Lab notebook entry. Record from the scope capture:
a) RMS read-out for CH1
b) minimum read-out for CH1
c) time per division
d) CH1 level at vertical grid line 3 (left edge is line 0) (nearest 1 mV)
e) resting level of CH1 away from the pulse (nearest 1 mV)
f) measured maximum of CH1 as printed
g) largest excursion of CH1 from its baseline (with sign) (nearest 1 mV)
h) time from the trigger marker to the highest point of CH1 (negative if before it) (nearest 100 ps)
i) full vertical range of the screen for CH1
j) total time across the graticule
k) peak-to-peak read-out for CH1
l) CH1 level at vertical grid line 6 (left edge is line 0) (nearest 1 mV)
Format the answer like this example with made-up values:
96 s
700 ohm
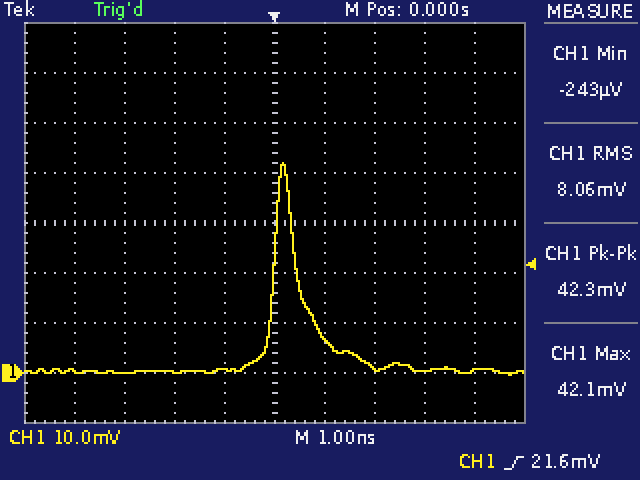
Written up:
8.06 mV
-243 µV
1 ns
0 mV
0 mV
42.1 mV
+42 mV
+200 ps
80 mV
10 ns
42.3 mV
7 mV
